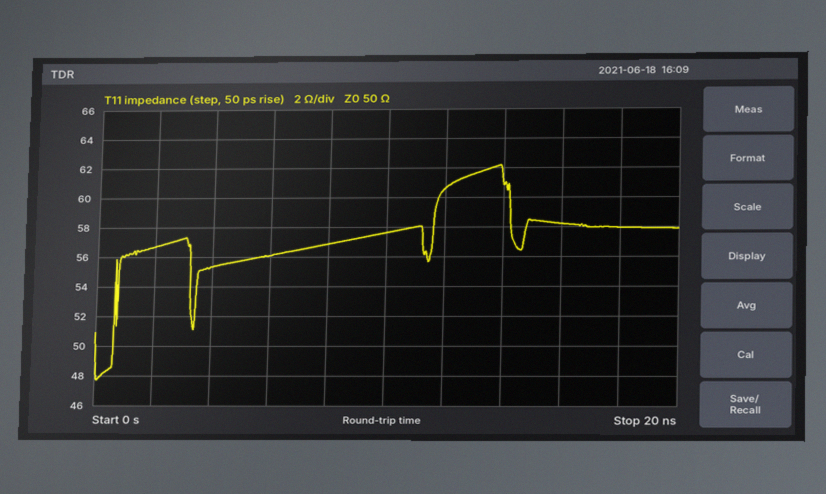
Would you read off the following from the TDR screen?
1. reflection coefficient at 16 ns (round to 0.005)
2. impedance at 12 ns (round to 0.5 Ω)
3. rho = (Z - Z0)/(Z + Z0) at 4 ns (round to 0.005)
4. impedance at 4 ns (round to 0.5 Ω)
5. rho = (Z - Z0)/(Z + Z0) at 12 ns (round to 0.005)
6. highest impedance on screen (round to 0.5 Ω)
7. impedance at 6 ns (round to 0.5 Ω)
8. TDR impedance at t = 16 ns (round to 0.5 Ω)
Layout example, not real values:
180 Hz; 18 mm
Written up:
+0.075; 60.5 Ω; +0.050; 55.5 Ω; +0.095; 62.0 Ω; 56.0 Ω; 58.0 Ω
